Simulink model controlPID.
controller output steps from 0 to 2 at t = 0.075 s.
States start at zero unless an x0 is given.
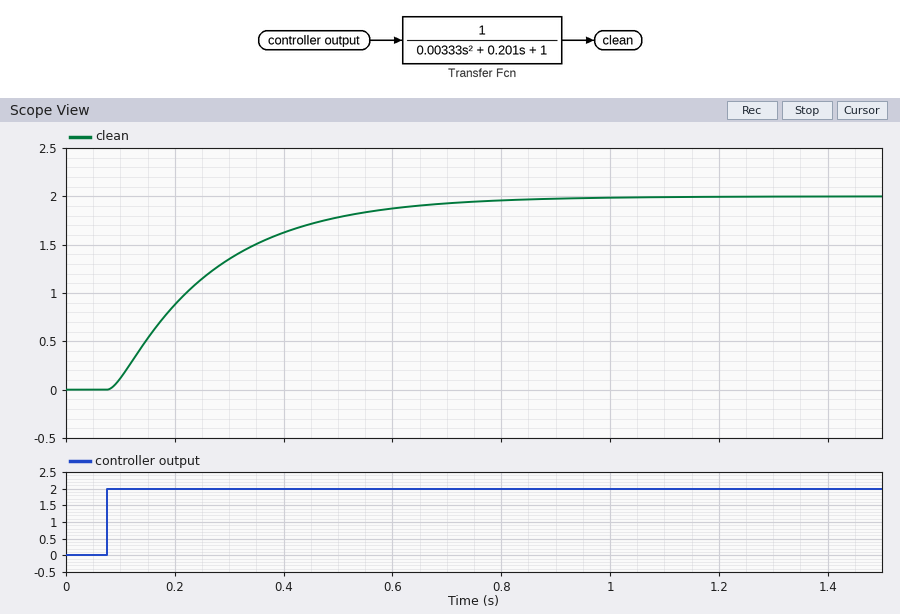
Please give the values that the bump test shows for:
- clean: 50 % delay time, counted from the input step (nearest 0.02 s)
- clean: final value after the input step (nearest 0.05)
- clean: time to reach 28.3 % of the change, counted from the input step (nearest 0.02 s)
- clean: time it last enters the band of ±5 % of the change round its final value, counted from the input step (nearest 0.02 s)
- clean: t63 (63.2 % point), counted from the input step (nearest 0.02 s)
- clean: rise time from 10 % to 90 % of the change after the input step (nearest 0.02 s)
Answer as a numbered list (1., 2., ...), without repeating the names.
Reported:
1. 0.14 s
2. 2.00
3. 0.08 s
4. 0.56 s
5. 0.20 s
6. 0.40 s
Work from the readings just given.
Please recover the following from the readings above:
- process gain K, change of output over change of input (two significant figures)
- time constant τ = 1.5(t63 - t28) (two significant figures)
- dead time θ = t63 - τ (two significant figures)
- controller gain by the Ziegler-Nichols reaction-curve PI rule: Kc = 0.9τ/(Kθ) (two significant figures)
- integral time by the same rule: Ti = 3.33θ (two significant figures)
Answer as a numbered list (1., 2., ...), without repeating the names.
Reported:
1. 1.0
2. 0.18 s
3. 0.020 s
4. 8.1
5. 0.067 s
